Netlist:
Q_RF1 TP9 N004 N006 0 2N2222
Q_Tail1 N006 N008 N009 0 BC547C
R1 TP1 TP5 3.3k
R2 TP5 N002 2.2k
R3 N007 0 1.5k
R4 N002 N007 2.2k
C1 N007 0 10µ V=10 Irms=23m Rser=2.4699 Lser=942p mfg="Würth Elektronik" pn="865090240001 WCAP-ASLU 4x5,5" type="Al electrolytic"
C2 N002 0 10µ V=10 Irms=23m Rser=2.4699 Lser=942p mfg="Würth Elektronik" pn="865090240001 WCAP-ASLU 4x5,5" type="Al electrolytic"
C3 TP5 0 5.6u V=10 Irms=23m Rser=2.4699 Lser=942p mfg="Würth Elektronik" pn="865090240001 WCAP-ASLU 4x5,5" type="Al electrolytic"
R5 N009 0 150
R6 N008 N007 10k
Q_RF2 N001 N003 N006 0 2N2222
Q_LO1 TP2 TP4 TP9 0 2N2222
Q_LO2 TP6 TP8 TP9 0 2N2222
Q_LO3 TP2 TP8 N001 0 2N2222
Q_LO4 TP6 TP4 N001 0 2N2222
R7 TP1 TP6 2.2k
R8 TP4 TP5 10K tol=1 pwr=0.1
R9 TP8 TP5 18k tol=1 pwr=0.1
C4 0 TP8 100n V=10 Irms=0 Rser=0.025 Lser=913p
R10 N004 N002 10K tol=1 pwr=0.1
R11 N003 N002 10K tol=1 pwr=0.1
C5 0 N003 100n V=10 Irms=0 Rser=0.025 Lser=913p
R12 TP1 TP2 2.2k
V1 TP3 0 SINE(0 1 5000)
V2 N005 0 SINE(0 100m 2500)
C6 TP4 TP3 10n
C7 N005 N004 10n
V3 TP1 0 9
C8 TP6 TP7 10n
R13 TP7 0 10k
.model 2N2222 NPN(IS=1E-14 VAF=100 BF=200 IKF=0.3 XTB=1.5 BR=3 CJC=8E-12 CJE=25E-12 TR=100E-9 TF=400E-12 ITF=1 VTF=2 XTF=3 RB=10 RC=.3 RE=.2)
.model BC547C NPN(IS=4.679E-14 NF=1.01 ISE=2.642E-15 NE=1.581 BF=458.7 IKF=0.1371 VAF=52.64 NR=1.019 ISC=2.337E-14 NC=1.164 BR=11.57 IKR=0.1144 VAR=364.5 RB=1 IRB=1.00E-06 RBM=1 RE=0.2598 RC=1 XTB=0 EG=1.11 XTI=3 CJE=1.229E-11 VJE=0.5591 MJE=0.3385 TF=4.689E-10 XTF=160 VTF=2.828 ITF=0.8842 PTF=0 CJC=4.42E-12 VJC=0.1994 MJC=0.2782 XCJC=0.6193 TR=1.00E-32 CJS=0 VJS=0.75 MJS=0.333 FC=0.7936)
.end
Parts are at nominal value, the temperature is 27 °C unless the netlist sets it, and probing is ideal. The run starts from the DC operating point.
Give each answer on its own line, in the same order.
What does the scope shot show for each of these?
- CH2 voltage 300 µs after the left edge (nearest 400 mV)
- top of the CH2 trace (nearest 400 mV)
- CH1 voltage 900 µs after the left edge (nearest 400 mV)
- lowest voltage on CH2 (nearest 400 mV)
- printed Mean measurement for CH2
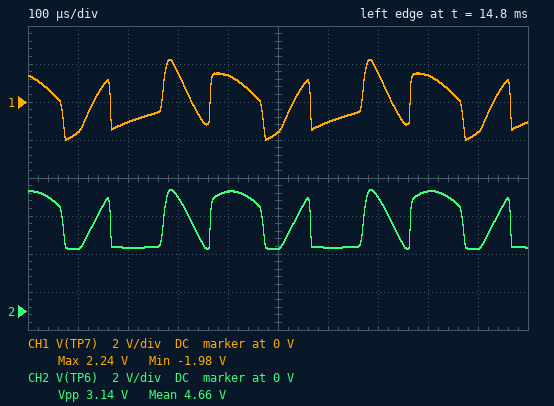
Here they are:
6.0 V
6.4 V
-1.6 V
3.2 V
4.66 V
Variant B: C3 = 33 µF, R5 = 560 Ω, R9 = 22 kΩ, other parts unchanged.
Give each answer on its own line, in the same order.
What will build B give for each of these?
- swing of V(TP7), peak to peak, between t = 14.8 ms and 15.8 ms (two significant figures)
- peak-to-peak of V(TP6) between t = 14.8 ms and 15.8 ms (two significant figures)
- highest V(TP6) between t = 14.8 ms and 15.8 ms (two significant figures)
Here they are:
2.9 V
2.4 V
8.7 V
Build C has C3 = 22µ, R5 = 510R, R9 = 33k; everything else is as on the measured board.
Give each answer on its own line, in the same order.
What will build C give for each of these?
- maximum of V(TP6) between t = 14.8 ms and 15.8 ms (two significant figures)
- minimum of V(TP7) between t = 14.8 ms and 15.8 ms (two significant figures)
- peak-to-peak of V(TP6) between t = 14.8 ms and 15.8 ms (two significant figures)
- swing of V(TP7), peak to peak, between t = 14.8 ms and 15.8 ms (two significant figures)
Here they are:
8.6 V
-1.6 V
2.6 V
3.1 V
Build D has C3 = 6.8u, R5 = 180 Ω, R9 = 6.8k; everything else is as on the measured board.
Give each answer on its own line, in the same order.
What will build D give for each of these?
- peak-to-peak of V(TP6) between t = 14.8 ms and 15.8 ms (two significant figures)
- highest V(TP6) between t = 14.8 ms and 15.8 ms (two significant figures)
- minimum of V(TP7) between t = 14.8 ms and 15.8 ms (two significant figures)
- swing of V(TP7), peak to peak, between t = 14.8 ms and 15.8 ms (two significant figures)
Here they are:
3.2 V
7.1 V
-1.7 V
3.9 V
